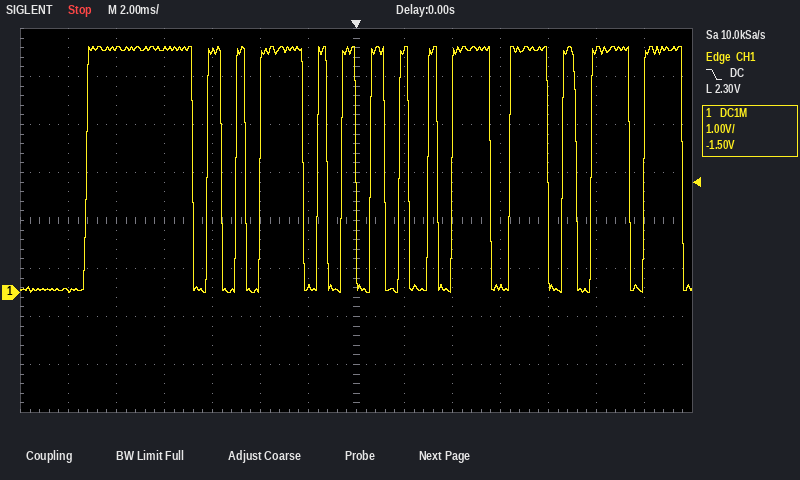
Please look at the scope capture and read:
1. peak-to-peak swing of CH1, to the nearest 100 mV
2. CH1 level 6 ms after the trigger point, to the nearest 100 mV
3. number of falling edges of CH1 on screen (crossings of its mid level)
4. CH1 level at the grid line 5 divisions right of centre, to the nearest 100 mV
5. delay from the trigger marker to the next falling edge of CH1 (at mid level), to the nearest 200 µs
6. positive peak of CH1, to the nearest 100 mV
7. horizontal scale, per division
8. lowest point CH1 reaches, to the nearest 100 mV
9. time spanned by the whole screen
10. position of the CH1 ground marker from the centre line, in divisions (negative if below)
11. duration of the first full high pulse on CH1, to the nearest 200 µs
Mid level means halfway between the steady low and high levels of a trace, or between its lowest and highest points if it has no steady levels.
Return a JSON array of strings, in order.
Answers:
["5.1 V", "100 mV", "14", "5.0 V", "1.2 ms", "5.1 V", "2 ms", "0.0 V", "28 ms", "-1.5 div", "4.4 ms"]
